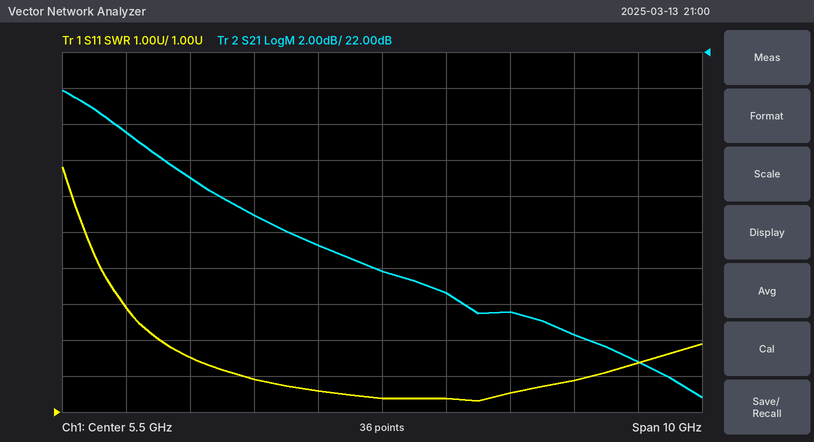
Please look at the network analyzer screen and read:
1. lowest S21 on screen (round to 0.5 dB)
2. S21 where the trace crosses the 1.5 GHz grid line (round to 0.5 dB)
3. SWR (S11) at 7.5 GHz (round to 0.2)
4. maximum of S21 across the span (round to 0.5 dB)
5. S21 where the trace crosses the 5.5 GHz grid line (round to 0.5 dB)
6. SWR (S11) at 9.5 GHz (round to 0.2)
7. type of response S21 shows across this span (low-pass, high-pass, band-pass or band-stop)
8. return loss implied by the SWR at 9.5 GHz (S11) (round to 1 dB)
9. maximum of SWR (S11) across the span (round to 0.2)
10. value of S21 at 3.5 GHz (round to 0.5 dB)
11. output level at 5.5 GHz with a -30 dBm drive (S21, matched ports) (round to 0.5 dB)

3.0 dB
17.5 dB
1.6
20.0 dB
10.0 dB
2.4
low-pass
8 dB
7.8
13.0 dB
-20.0 dBm
